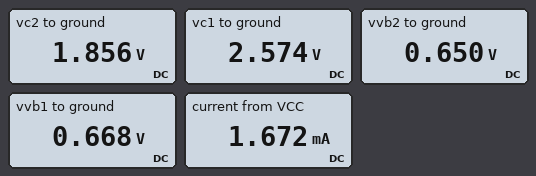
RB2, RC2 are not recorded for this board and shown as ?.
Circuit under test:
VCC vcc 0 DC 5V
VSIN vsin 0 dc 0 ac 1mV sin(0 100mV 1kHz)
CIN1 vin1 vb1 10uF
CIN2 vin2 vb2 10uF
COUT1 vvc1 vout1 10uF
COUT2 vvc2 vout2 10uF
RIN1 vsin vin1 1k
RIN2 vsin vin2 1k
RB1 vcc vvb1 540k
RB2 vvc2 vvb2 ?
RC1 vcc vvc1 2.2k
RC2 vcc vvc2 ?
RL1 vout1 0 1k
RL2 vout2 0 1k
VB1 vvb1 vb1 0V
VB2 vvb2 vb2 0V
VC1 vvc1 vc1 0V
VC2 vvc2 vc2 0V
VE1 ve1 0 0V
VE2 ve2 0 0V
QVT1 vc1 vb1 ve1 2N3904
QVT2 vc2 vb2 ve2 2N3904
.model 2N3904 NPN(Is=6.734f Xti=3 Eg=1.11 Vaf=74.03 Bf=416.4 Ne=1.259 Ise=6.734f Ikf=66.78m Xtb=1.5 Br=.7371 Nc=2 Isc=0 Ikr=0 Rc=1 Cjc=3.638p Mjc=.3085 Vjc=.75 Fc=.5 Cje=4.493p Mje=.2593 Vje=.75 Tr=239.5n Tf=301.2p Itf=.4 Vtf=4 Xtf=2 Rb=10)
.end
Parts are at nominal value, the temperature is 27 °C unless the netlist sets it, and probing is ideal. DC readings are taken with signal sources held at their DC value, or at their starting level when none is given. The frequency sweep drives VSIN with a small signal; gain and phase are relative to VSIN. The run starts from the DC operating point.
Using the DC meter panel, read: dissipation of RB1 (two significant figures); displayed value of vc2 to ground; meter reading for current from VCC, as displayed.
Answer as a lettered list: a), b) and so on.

a) 35 µW
b) 1.856 V
c) 1.672 mA
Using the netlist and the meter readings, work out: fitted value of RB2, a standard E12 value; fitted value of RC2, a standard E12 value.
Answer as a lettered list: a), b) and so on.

a) 270 kΩ
b) 5.6 kΩ
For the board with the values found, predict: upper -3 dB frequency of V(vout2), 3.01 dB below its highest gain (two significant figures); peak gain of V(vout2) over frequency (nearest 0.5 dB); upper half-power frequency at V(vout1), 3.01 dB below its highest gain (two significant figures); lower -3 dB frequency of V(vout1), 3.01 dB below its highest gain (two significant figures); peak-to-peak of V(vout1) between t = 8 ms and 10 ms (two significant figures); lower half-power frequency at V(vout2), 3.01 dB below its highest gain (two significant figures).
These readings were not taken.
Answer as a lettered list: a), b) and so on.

a) 2.9 MHz
b) 23.5 dB
c) 2.1 MHz
d) 6.6 Hz
e) 2.9 V
f) 4.3 Hz
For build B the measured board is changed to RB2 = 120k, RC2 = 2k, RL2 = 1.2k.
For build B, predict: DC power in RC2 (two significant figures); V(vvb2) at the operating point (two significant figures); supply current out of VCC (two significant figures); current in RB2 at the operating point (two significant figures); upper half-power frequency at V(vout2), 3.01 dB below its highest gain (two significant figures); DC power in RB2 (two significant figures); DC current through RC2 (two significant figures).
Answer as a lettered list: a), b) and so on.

a) 4.6 mW
b) 680 mV
c) 2.6 mA
d) 11 µA
e) 1.9 MHz
f) 14 µW
g) 1.5 mA
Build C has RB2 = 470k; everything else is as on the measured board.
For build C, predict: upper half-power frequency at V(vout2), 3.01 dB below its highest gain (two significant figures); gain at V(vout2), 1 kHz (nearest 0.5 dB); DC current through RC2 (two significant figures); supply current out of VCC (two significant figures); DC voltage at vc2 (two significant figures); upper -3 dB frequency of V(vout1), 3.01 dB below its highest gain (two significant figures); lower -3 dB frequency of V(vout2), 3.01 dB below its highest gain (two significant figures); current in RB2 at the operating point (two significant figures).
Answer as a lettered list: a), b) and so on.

a) 3.4 MHz
b) 22.0 dB
c) 460 µA
d) 1.6 mA
e) 2.4 V
f) 2.1 MHz
g) 3.6 Hz
h) 3.8 µA
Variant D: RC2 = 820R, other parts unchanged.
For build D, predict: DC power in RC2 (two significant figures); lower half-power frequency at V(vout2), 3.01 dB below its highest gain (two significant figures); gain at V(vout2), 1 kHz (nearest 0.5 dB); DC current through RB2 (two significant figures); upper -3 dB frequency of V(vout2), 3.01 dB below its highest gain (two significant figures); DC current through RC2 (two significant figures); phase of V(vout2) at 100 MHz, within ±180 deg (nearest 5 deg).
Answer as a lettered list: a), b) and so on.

a) 2.2 mW
b) 11 Hz
c) 25.5 dB
d) 11 µA
e) 2.6 MHz
f) 1.6 mA
g) 80 deg
